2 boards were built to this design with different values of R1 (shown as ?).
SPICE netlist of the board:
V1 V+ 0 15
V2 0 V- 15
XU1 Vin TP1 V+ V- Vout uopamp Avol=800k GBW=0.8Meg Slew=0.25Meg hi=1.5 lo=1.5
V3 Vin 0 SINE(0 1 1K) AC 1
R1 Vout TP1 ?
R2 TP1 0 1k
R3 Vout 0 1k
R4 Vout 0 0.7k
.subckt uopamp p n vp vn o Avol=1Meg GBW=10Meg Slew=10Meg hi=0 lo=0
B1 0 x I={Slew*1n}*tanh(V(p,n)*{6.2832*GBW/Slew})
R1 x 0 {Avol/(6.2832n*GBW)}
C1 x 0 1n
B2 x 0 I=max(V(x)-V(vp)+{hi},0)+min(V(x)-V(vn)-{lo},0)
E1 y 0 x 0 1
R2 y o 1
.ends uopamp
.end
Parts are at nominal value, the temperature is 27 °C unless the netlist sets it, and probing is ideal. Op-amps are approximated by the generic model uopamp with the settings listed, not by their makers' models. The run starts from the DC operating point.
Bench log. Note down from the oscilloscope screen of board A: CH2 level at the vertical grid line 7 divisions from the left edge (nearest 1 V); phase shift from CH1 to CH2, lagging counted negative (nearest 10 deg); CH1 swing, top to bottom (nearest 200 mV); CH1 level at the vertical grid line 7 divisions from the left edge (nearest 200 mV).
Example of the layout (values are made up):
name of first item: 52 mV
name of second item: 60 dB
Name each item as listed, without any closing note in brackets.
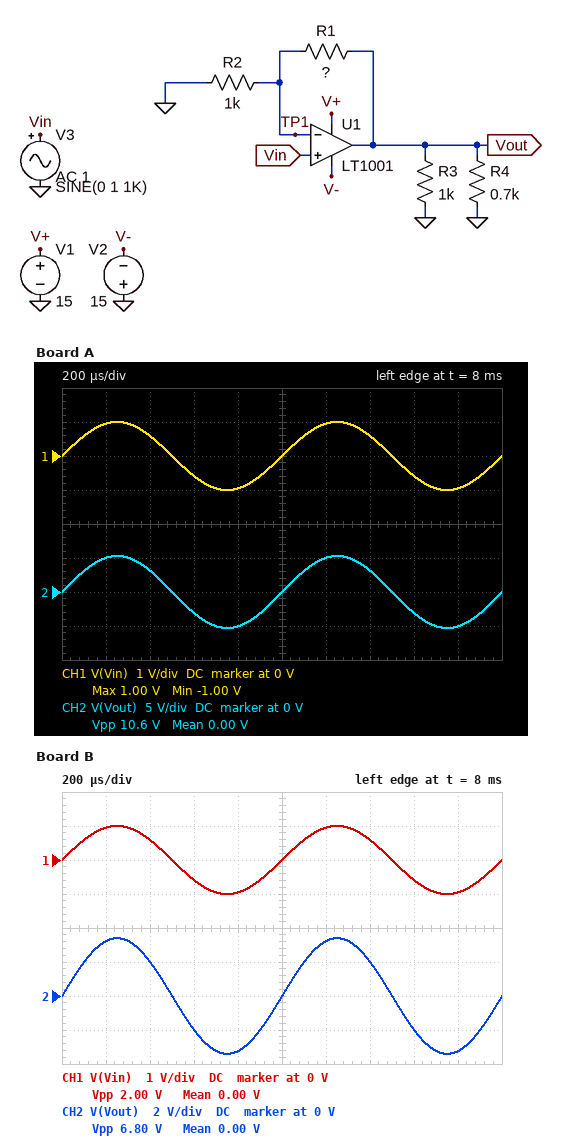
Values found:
CH2 level at the vertical grid line 7 divisions from the left edge: 3 V
phase shift from CH1 to CH2, lagging counted negative: 0 deg
CH1 swing, top to bottom: 2.0 V
CH1 level at the vertical grid line 7 divisions from the left edge: 600 mV
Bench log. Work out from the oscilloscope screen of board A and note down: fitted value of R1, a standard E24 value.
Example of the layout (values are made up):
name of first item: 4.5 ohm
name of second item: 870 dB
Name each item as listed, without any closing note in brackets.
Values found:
fitted value of R1, a standard E24 value: 4.3 kΩ
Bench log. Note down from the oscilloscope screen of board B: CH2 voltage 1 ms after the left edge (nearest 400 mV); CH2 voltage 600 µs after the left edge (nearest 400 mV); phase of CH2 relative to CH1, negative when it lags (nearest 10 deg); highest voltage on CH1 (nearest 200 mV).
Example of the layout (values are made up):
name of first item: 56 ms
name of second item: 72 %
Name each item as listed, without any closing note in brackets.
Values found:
CH2 voltage 1 ms after the left edge: 0 V
CH2 voltage 600 µs after the left edge: -2.0 V
phase of CH2 relative to CH1, negative when it lags: 0 deg
highest voltage on CH1: 1.0 V
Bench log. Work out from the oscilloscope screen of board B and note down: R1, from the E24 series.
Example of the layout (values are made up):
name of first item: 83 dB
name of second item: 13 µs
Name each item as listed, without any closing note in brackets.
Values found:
R1, from the E24 series: 2.4 kΩ
